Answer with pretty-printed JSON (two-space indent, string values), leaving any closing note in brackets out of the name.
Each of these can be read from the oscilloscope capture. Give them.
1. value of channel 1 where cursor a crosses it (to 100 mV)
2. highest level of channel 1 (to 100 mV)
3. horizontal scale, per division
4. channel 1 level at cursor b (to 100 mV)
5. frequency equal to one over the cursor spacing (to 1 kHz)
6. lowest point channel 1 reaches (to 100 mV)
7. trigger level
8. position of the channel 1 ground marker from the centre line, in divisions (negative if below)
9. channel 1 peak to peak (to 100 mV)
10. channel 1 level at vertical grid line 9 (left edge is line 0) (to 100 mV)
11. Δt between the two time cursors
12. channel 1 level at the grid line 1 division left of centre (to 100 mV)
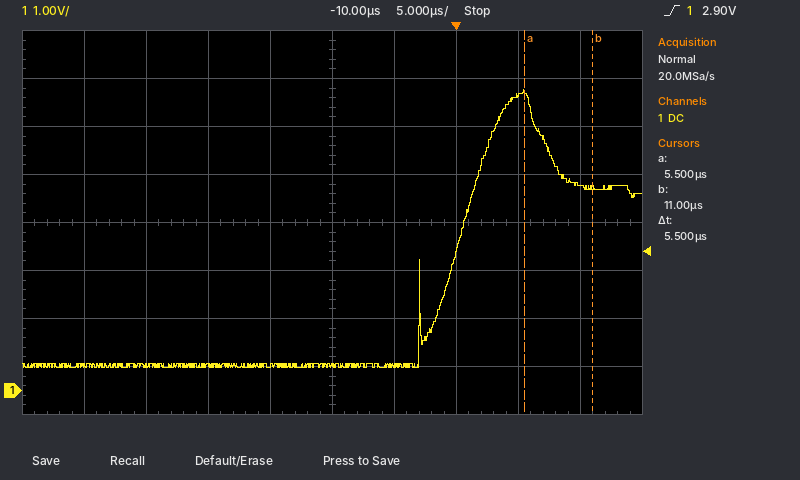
{
  "value of channel 1 where cursor a crosses it": "6.2 V",
  "highest level of channel 1": "6.3 V",
  "horizontal scale, per division": "5 µs",
  "channel 1 level at cursor b": "4.2 V",
  "frequency equal to one over the cursor spacing": "182 kHz",
  "lowest point channel 1 reaches": "500 mV",
  "trigger level": "2.90 V",
  "position of the channel 1 ground marker from the centre line, in divisions": "-3.5 div",
  "channel 1 peak to peak": "5.8 V",
  "channel 1 level at vertical grid line 9 (left edge is line 0)": "4.3 V",
  "Δt between the two time cursors": "5.5 µs",
  "channel 1 level at the grid line 1 division left of centre": "500 mV"
}
